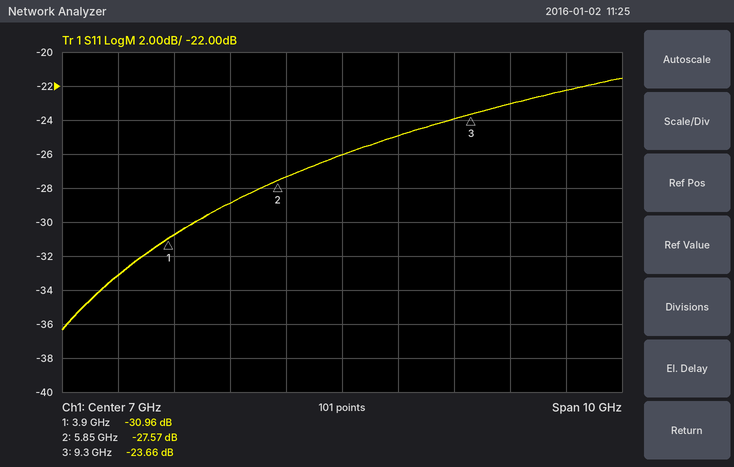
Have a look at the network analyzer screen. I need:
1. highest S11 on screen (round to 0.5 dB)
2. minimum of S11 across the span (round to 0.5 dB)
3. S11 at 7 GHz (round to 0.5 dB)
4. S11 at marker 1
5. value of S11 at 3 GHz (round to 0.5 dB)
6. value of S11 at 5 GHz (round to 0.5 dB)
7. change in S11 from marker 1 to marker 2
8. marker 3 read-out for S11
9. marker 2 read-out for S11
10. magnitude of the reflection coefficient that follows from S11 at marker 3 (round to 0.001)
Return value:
-21.5 dB
-36.5 dB
-26.0 dB
-30.96 dB
-33.0 dB
-29.0 dB
3.39 dB
-23.66 dB
-27.57 dB
0.066
